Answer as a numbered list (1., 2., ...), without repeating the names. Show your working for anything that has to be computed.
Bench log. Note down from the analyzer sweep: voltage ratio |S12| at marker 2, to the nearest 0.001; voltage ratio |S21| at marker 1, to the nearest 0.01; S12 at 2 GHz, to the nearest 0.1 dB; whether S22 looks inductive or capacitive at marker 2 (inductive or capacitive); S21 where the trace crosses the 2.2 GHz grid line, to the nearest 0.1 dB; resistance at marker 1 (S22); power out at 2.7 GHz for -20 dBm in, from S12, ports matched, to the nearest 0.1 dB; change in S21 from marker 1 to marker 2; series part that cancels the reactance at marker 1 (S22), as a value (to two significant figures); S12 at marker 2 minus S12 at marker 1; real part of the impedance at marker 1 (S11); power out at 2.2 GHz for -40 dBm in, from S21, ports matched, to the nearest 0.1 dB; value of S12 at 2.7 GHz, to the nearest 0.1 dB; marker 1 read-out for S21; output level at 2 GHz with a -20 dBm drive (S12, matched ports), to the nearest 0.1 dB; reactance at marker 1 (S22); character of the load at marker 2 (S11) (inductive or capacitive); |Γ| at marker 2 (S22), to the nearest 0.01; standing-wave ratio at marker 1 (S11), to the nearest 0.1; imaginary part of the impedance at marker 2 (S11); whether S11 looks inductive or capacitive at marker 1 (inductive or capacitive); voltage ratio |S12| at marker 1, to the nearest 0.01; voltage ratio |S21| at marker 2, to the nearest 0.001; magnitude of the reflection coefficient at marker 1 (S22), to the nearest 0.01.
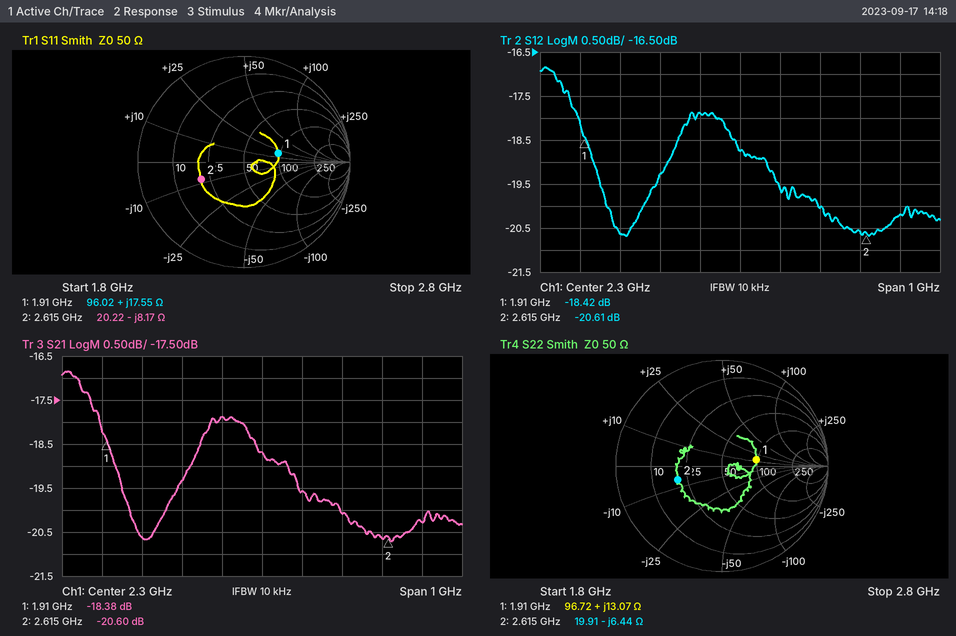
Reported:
1. 10^(-20.61/20) ≈ 0.093
2. 10^(-18.38/20) ≈ 0.12
3. -20.6 dB
4. capacitive
5. -17.9 dB
6. 96.72 Ω
7. -20 dBm + (-20.2 dB) = -40.2 dBm
8. -20.6 − (-18.38) = -2.22 dB
9. C = 1/(2π × 1.91 GHz × 13.07 Ω) ≈ 6.4 pF
10. -20.61 − (-18.42) = -2.19 dB
11. 96.02 Ω
12. -40 dBm + (-17.9 dB) = -57.9 dBm
13. -20.2 dB
14. -18.38 dB
15. -20 dBm + (-20.6 dB) = -40.6 dBm
16. +13.07 Ω
17. capacitive
18. 0.44
19. 2.0
20. -8.17 Ω
21. inductive
22. 10^(-18.42/20) ≈ 0.12
23. 10^(-20.6/20) ≈ 0.093
24. 0.33
